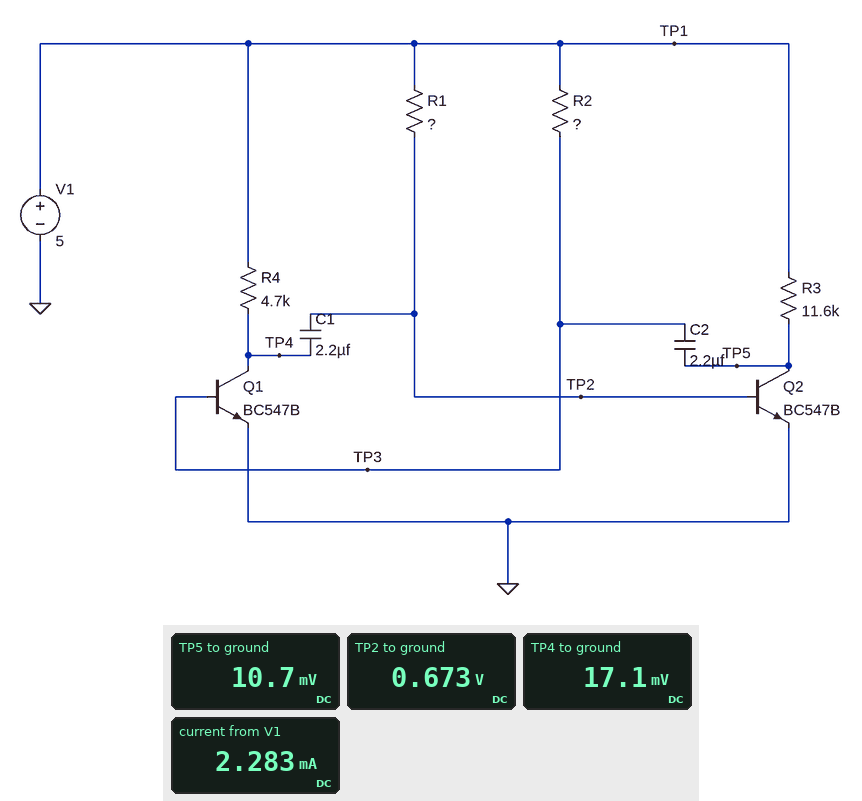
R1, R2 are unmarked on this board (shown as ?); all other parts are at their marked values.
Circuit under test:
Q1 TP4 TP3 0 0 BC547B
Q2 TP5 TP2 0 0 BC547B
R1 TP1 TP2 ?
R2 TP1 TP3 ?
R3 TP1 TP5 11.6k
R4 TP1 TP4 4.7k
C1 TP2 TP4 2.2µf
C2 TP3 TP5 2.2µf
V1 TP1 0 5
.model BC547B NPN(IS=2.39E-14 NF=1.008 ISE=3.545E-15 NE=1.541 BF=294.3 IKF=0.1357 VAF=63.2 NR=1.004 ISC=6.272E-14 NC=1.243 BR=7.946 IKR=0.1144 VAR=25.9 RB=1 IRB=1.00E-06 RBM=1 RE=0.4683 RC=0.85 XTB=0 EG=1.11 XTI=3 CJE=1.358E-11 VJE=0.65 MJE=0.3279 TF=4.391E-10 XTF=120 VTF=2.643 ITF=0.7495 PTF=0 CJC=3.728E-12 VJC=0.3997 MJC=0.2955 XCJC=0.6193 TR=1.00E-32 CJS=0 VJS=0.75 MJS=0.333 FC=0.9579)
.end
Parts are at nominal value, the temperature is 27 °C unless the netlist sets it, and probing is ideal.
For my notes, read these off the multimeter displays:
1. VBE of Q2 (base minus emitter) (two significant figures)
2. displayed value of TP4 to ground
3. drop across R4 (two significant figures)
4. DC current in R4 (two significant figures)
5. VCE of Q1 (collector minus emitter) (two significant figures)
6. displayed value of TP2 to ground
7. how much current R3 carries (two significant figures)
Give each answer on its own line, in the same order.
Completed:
670 mV
17.1 mV
5.0 V
1.1 mA
17 mV
0.673 V
430 µA
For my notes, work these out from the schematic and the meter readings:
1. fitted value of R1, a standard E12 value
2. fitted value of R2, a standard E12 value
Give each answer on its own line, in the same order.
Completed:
10 kΩ
12 kΩ
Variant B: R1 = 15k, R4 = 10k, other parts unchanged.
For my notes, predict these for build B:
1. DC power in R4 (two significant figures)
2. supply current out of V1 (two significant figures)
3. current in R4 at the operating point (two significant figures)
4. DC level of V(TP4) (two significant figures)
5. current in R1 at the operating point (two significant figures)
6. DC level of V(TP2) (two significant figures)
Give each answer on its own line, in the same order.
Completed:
2.5 mW
1.6 mA
500 µA
12 mV
290 µA
660 mV
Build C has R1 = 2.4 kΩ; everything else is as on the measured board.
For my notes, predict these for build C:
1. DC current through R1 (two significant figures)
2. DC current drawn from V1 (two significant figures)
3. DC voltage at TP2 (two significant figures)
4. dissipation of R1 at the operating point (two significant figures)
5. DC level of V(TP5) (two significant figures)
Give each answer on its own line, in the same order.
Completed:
1.8 mA
3.6 mA
710 mV
7.7 mW
9.3 mV
